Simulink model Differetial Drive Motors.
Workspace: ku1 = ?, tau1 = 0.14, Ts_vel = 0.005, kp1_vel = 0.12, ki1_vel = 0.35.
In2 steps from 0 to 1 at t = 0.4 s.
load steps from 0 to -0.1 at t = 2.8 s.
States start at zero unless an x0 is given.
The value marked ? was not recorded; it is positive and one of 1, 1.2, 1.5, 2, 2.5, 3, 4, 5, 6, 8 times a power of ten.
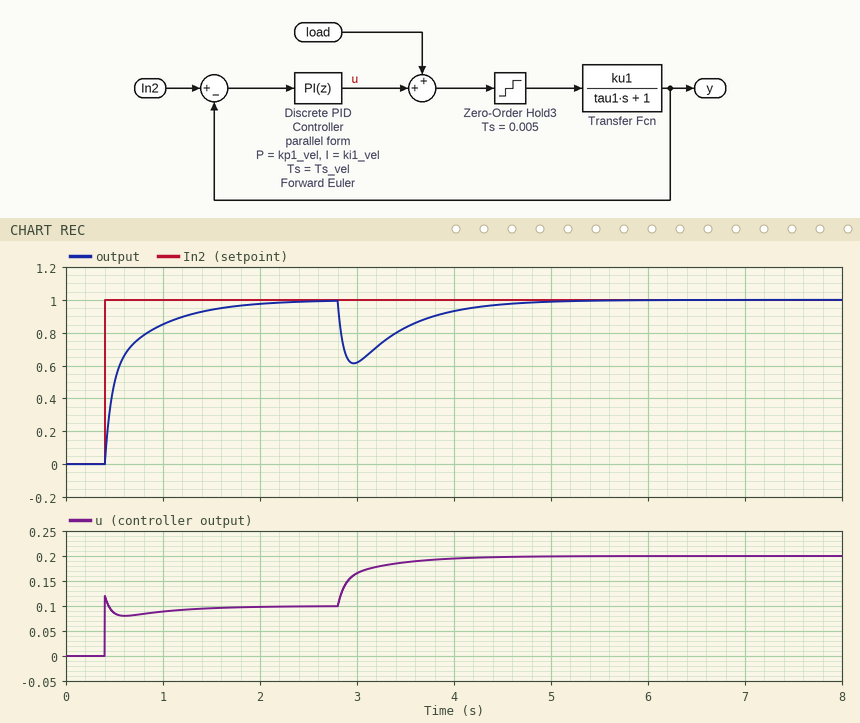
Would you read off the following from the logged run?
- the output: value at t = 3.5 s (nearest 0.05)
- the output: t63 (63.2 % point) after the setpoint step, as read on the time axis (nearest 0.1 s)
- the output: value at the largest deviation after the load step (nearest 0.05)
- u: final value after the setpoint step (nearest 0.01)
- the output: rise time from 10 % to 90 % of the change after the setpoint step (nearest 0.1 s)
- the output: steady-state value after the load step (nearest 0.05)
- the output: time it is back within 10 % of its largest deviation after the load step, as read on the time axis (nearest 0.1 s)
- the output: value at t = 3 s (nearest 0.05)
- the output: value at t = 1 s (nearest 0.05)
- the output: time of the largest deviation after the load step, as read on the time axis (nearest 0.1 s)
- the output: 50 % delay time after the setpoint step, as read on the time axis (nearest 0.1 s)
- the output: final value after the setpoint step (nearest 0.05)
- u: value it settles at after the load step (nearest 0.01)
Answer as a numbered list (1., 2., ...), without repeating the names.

1. 0.85
2. 0.6 s
3. 0.60
4. 0.10
5. 0.8 s
6. 1.00
7. 4.3 s
8. 0.60
9. 0.85
10. 3.0 s
11. 0.5 s
12. 1.00
13. 0.20
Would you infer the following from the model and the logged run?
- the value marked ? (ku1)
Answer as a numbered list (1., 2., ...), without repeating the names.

1. 10
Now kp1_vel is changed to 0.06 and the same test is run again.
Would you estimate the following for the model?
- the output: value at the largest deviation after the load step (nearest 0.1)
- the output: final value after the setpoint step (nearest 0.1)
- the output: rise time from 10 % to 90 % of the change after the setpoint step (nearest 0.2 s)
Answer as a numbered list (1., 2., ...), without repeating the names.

1. 0.5
2. 1.0
3. 0.6 s
